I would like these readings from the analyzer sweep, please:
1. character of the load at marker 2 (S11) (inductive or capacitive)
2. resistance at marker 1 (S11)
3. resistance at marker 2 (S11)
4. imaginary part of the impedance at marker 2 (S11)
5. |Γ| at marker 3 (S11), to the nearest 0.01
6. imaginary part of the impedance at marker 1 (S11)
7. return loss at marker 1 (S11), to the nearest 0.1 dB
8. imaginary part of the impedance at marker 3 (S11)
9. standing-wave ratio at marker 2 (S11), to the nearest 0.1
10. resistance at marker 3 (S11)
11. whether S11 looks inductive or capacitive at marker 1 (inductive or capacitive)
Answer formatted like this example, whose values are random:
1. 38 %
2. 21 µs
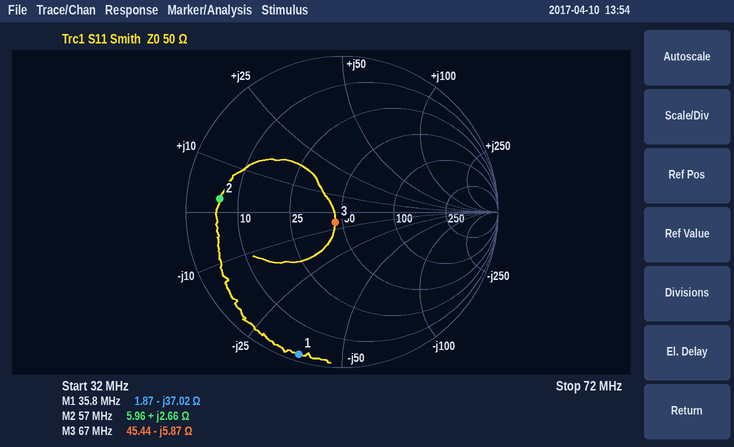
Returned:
1. inductive
2. 1.87 Ω
3. 5.96 Ω
4. +2.66 Ω
5. 0.08
6. -37.02 Ω
7. 0.4 dB
8. -5.87 Ω
9. 8.4
10. 45.44 Ω
11. capacitive
